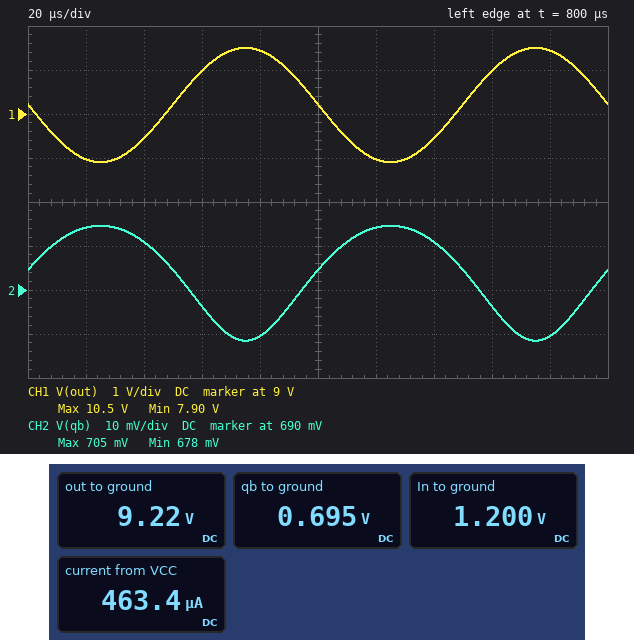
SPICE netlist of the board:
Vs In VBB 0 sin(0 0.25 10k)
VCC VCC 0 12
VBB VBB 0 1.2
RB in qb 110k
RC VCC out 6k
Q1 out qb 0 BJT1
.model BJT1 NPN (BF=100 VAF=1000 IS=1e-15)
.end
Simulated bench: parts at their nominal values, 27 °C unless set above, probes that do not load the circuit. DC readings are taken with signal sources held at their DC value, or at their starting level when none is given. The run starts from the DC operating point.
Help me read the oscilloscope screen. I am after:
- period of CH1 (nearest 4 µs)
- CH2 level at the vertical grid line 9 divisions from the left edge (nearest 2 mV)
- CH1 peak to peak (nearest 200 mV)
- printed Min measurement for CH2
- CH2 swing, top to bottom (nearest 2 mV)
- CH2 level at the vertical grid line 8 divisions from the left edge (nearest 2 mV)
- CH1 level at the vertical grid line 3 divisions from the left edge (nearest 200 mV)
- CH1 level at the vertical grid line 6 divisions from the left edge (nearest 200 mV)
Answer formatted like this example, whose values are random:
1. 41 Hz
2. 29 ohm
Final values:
1. 100 µs
2. 680 mV
3. 2.6 V
4. 678 mV
5. 26 mV
6. 686 mV
7. 10.0 V
8. 8.0 V
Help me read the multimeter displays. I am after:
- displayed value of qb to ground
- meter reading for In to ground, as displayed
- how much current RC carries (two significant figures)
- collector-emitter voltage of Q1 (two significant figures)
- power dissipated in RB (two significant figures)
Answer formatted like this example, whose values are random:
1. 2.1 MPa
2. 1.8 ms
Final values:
1. 0.695 V
2. 1.200 V
3. 460 µA
4. 9.2 V
5. 2.3 µW
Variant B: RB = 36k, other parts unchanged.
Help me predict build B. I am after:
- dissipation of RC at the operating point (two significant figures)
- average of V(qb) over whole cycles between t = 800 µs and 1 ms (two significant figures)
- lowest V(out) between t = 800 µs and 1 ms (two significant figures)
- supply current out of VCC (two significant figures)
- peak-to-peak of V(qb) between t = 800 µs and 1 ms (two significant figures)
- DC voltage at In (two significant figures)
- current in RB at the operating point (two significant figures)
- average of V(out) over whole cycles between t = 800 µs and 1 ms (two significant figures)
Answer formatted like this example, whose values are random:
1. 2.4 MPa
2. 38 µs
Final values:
1. 11 mW
2. 720 mV
3. 230 mV
4. 1.3 mA
5. 27 mV
6. 1.2 V
7. 13 µA
8. 4.0 V
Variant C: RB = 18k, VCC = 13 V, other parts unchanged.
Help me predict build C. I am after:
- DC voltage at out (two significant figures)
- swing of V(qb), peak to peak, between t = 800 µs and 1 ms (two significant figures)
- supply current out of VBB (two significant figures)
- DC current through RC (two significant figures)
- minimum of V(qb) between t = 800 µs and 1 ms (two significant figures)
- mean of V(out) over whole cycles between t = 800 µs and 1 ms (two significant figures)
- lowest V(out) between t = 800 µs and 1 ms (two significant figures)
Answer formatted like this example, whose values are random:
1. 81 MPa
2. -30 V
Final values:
1. 160 mV
2. 14 mV
3. 26 µA
4. 2.1 mA
5. 720 mV
6. 1.5 V
7. 120 mV
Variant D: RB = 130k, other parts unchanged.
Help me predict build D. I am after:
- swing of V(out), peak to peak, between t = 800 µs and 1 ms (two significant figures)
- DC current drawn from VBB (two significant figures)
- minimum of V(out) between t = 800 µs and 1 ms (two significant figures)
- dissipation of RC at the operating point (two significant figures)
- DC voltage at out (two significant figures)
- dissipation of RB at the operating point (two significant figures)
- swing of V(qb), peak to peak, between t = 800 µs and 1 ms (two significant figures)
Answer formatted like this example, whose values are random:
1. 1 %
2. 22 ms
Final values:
1. 2.2 V
2. 3.9 µA
3. 8.5 V
4. 940 µW
5. 9.6 V
6. 2.0 µW
7. 26 mV
